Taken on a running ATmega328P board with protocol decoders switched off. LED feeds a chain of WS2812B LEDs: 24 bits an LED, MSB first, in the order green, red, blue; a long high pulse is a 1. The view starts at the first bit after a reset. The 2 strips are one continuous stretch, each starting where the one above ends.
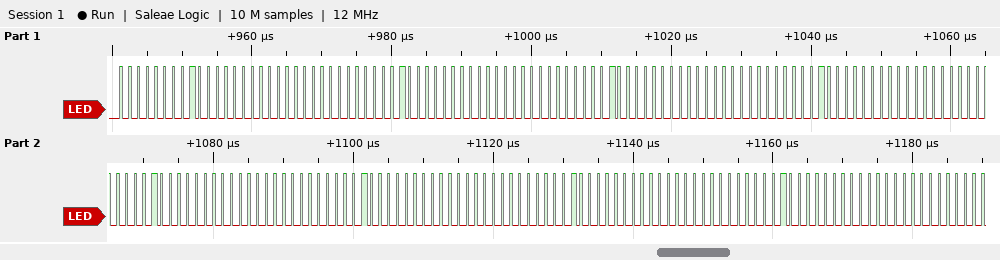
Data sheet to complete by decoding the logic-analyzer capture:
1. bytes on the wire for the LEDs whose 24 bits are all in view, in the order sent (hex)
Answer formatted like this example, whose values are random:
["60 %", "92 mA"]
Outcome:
["00 80 00 00 80 00 00 80 00 00 80 00 00 80 00 00 80 00 00 80 00 00 80 00"]
